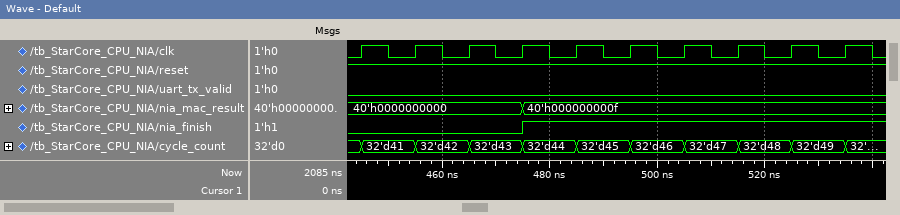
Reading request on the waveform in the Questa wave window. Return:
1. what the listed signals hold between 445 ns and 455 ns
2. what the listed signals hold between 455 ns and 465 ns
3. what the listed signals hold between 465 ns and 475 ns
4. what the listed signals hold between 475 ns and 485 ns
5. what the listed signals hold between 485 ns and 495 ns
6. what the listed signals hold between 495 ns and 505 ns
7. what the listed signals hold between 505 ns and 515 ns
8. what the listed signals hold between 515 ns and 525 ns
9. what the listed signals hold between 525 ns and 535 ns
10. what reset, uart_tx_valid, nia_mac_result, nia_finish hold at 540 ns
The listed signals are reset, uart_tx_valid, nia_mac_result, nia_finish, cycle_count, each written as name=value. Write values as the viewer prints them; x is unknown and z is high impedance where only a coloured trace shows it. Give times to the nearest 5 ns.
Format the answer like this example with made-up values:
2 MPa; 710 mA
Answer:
reset=1, uart_tx_valid=0, nia_mac_result=40'h0000000000, nia_finish=0, cycle_count=32'd41; reset=1, uart_tx_valid=0, nia_mac_result=40'h0000000000, nia_finish=0, cycle_count=32'd42; reset=1, uart_tx_valid=0, nia_mac_result=40'h0000000000, nia_finish=0, cycle_count=32'd43; reset=1, uart_tx_valid=0, nia_mac_result=40'h000000000f, nia_finish=1, cycle_count=32'd44; reset=1, uart_tx_valid=0, nia_mac_result=40'h000000000f, nia_finish=1, cycle_count=32'd45; reset=1, uart_tx_valid=0, nia_mac_result=40'h000000000f, nia_finish=1, cycle_count=32'd46; reset=1, uart_tx_valid=0, nia_mac_result=40'h000000000f, nia_finish=1, cycle_count=32'd47; reset=1, uart_tx_valid=0, nia_mac_result=40'h000000000f, nia_finish=1, cycle_count=32'd48; reset=1, uart_tx_valid=0, nia_mac_result=40'h000000000f, nia_finish=1, cycle_count=32'd49; reset=1, uart_tx_valid=0, nia_mac_result=40'h000000000f, nia_finish=1
